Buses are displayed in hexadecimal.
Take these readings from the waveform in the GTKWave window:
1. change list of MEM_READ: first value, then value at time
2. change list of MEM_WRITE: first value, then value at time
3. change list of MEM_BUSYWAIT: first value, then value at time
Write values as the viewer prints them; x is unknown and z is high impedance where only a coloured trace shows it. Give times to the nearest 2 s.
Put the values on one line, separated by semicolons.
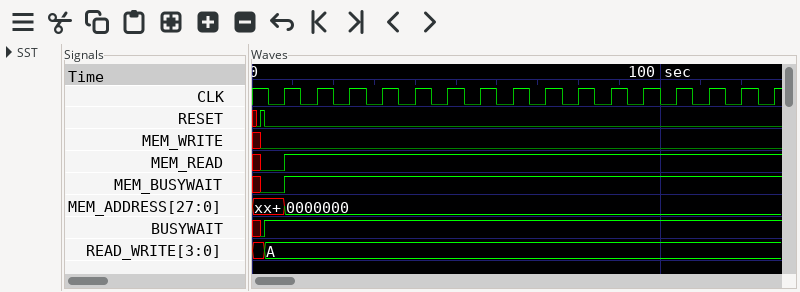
x, 0 at 2 s, 1 at 8 s; x, 0 at 2 s; x, 0 at 2 s, 1 at 8 s
